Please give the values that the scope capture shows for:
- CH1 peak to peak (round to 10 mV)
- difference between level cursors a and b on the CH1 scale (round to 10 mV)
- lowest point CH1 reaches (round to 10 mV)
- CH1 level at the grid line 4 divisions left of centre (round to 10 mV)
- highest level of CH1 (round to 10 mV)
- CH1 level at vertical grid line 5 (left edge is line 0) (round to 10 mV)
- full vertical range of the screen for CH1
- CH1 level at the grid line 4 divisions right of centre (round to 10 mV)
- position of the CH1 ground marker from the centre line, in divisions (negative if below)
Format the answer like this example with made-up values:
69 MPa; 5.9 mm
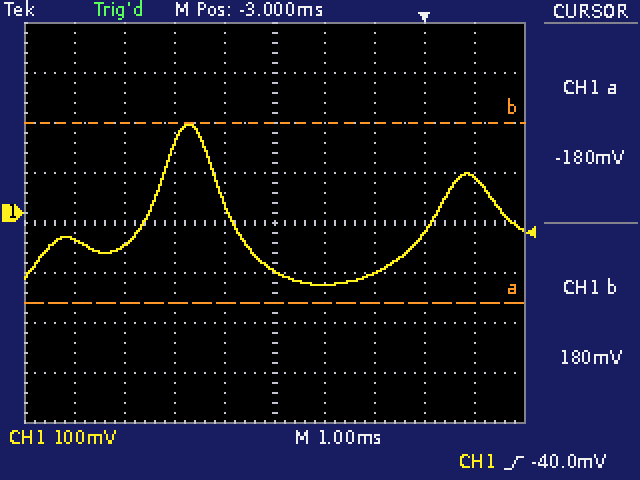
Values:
320 mV; 360 mV; -140 mV; -50 mV; 180 mV; -120 mV; 800 mV; 70 mV; +0.2 div
